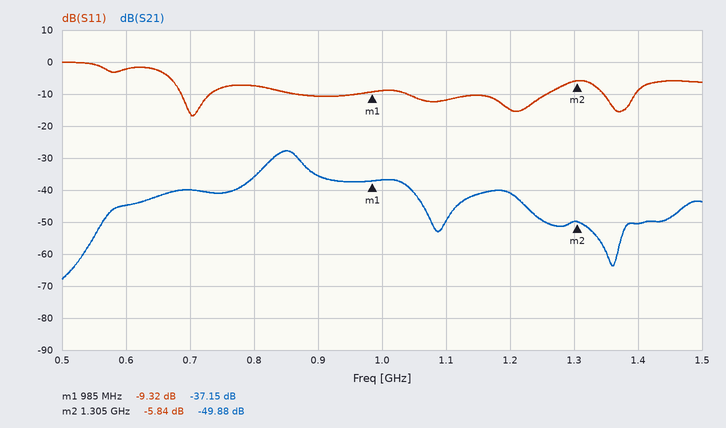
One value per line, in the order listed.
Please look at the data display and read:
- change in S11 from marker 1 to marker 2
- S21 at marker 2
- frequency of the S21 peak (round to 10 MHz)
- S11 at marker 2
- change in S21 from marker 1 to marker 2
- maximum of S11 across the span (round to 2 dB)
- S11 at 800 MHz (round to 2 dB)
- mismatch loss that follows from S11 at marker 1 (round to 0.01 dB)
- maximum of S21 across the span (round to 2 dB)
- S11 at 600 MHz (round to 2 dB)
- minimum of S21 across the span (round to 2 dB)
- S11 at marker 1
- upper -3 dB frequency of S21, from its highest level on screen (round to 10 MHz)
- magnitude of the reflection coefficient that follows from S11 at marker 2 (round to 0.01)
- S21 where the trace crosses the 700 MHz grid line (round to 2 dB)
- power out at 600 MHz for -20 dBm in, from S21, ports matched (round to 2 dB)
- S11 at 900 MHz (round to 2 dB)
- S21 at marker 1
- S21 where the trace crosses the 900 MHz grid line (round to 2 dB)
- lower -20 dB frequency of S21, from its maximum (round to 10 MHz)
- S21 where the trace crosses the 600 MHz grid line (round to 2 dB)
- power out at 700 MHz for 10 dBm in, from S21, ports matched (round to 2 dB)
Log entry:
3.48 dB
-49.88 dB
850 MHz
-5.84 dB
-12.73 dB
0 dB
-8 dB
0.54 dB
-28 dB
-2 dB
-68 dB
-9.32 dB
870 MHz
0.51
-40 dB
-64 dBm
-10 dB
-37.15 dB
-36 dB
570 MHz
-44 dB
-30 dBm
